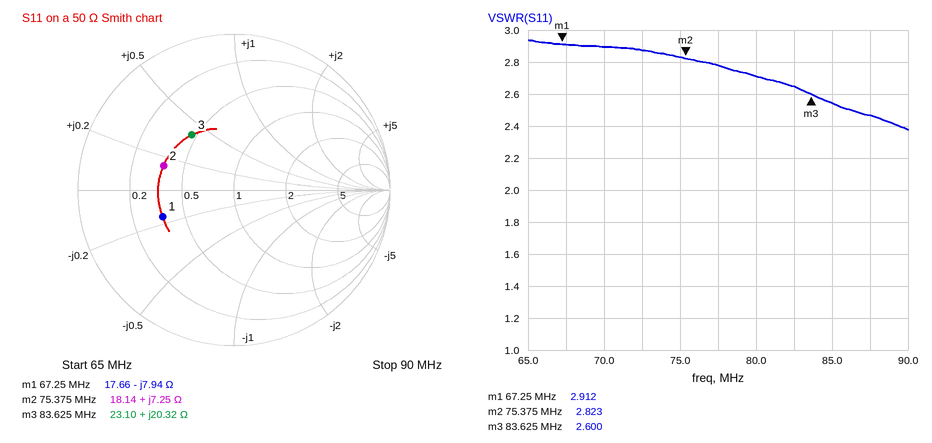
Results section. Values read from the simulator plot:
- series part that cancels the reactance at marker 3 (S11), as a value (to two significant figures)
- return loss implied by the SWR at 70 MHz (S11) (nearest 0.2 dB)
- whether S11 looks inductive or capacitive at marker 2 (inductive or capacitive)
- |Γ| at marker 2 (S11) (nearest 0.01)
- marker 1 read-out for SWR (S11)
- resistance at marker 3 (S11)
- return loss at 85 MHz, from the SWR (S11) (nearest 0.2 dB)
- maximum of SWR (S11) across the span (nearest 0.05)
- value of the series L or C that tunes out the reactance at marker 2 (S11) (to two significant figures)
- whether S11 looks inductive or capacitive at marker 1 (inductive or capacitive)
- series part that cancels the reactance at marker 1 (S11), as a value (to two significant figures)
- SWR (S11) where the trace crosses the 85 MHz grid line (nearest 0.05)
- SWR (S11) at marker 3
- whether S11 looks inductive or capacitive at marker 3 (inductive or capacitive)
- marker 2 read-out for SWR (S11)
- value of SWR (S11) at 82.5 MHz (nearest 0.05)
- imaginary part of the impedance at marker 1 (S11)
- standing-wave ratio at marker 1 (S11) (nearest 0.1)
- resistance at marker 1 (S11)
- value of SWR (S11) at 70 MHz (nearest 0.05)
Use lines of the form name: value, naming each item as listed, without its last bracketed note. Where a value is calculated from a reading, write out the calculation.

series part that cancels the reactance at marker 3 (S11), as a value: C = 1/(2π × 83.625 MHz × 20.32 Ω) ≈ 94 pF
return loss implied by the SWR at 70 MHz (S11): −20 log10((2.9 − 1)/(2.9 + 1)) ≈ 6.2 dB
whether S11 looks inductive or capacitive at marker 2: inductive
|Γ| at marker 2 (S11): 0.48
marker 1 read-out for SWR: 2.912
resistance at marker 3: 23.10 Ω
return loss at 85 MHz, from the SWR (S11): −20 log10((2.55 − 1)/(2.55 + 1)) ≈ 7.2 dB
maximum of SWR (S11) across the span: 2.95
value of the series L or C that tunes out the reactance at marker 2 (S11): C = 1/(2π × 75.375 MHz × 7.25 Ω) ≈ 291 pF, so 290 pF to two significant figures
whether S11 looks inductive or capacitive at marker 1: capacitive
series part that cancels the reactance at marker 1 (S11), as a value: L = 7.94 Ω/(2π × 67.25 MHz) ≈ 19 nH
SWR (S11) where the trace crosses the 85 MHz grid line: 2.55
SWR (S11) at marker 3: 2.600
whether S11 looks inductive or capacitive at marker 3: inductive
marker 2 read-out for SWR: 2.823
value of SWR (S11) at 82.5 MHz: 2.65
imaginary part of the impedance at marker 1: -7.94 Ω
standing-wave ratio at marker 1 (S11): 2.9
resistance at marker 1: 17.66 Ω
value of SWR (S11) at 70 MHz: 2.90
